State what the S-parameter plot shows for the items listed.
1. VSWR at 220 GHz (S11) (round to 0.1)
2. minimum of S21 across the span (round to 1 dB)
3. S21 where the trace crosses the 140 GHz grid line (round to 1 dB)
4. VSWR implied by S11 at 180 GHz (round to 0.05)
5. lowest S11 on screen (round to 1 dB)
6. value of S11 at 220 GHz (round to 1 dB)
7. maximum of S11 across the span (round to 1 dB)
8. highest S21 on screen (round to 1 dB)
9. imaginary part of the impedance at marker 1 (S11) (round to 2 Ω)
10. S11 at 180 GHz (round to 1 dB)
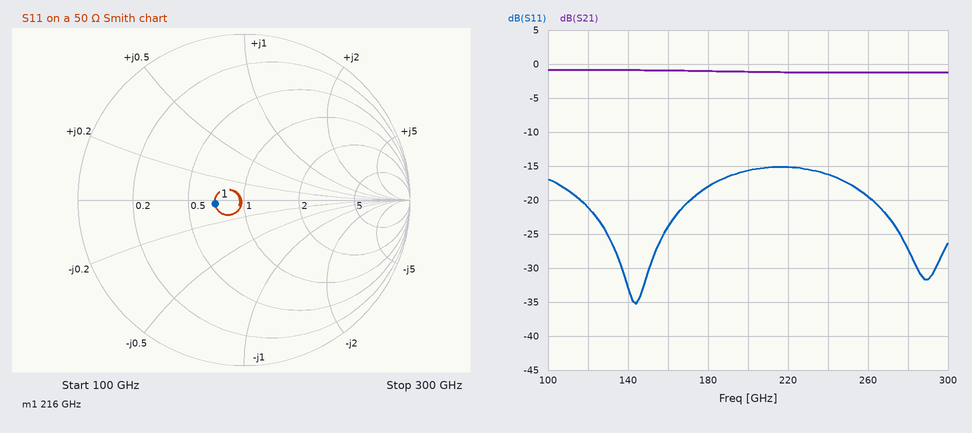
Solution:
1.4
-1 dB
-1 dB
1.30
-35 dB
-15 dB
-15 dB
-1 dB
-2 Ω
-18 dB
